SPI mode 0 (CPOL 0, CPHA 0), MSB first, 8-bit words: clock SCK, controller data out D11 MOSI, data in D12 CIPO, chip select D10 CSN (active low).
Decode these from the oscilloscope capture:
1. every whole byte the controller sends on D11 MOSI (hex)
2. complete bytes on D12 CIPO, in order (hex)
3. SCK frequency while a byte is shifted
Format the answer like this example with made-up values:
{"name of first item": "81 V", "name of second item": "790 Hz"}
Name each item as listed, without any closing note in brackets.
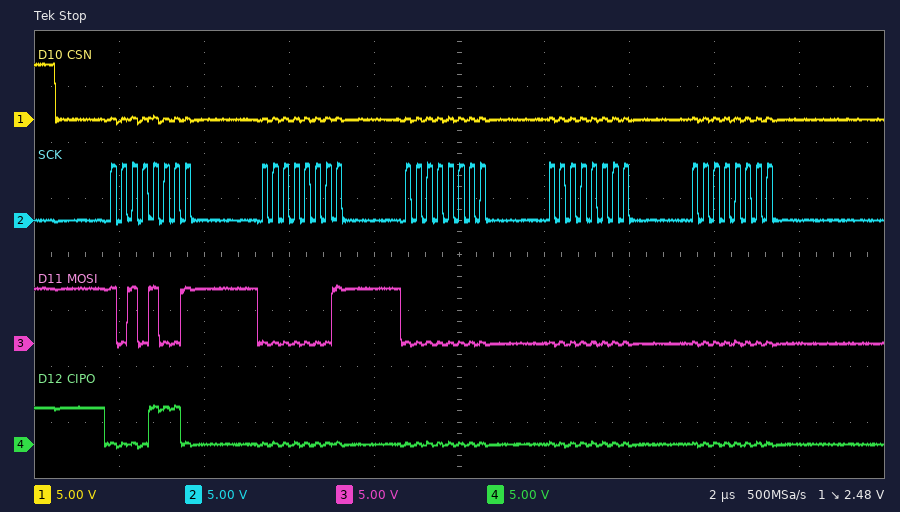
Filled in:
{"every whole byte the controller sends on D11 MOSI": "0xA9 0x01 0x00 0x00 0x00", "complete bytes on D12 CIPO, in order": "0x0E 0x00 0x00 0x00 0x00", "SCK frequency while a byte is shifted": "4 MHz"}
